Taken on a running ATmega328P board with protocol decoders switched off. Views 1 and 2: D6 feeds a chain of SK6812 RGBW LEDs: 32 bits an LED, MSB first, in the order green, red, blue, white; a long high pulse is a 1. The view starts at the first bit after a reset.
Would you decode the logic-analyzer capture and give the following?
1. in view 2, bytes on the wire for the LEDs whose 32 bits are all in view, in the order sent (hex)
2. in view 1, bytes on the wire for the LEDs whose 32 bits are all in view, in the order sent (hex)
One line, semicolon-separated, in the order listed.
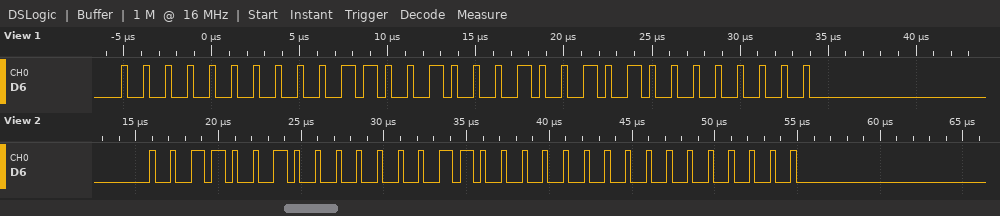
32 03 00 00; 00 32 25 00
